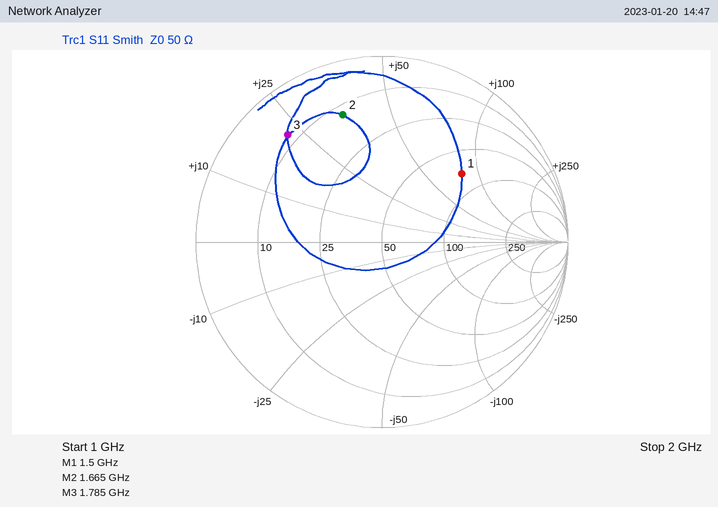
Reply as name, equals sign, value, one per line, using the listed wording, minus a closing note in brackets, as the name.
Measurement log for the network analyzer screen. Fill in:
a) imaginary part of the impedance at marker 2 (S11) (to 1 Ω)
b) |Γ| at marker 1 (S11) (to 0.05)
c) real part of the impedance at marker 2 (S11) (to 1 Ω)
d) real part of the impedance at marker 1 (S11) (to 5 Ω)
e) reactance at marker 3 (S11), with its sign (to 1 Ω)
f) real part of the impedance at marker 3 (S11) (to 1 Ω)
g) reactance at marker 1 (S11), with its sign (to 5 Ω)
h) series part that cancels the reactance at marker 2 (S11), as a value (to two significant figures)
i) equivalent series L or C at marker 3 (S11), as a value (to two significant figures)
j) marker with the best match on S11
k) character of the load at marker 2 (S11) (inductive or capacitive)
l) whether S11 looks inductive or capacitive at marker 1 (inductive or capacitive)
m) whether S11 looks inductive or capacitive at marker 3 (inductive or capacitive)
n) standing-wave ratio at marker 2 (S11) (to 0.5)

imaginary part of the impedance at marker 2 (S11) = +35 Ω
|Γ| at marker 1 (S11) = 0.55
real part of the impedance at marker 2 (S11) = 13 Ω
real part of the impedance at marker 1 (S11) = 75 Ω
reactance at marker 3 (S11), with its sign = +22 Ω
real part of the impedance at marker 3 (S11) = 8 Ω
reactance at marker 1 (S11), with its sign = +80 Ω
series part that cancels the reactance at marker 2 (S11), as a value = 2.7 pF
equivalent series L or C at marker 3 (S11), as a value = 2.0 nH
marker with the best match on S11 = marker 1
character of the load at marker 2 (S11) = inductive
whether S11 looks inductive or capacitive at marker 1 = inductive
whether S11 looks inductive or capacitive at marker 3 = inductive
standing-wave ratio at marker 2 (S11) = 6.0
